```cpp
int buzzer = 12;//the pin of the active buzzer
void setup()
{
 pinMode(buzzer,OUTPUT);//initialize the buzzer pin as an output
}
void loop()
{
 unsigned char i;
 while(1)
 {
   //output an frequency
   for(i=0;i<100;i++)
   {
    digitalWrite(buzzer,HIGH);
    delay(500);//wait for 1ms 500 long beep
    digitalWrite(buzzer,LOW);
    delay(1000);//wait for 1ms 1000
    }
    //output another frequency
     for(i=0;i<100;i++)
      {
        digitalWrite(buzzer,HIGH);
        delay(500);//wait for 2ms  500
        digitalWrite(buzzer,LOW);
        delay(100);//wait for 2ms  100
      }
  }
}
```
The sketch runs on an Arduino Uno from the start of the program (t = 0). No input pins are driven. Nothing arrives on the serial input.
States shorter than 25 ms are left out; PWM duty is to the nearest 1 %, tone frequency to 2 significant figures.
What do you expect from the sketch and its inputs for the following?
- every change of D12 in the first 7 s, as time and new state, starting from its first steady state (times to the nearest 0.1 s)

0 s high; 0.5 s low; 1.5 s high; 2 s low; 3 s high; 3.5 s low; 4.5 s high; 5 s low; 6 s high; 6.5 s low
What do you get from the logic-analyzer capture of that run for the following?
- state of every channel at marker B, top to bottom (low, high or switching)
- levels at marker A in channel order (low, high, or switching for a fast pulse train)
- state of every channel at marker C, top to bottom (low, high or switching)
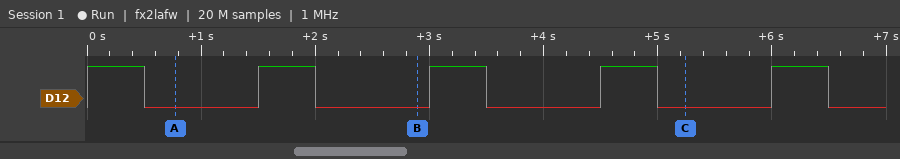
D12 low
D12 low
D12 low
